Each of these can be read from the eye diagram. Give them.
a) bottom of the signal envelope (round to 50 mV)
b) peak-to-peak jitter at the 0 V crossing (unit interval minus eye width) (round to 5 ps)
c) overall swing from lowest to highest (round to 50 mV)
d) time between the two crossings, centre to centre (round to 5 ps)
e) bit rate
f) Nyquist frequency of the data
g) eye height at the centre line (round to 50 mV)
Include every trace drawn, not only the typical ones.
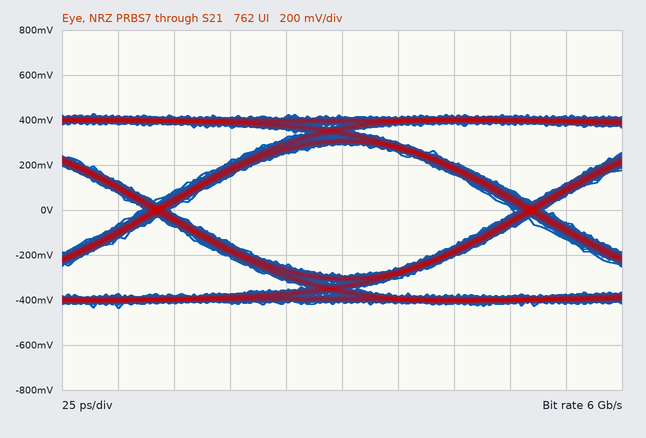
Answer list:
-450 mV
15 ps
850 mV
165 ps
6 Gb/s
3 GHz
600 mV
